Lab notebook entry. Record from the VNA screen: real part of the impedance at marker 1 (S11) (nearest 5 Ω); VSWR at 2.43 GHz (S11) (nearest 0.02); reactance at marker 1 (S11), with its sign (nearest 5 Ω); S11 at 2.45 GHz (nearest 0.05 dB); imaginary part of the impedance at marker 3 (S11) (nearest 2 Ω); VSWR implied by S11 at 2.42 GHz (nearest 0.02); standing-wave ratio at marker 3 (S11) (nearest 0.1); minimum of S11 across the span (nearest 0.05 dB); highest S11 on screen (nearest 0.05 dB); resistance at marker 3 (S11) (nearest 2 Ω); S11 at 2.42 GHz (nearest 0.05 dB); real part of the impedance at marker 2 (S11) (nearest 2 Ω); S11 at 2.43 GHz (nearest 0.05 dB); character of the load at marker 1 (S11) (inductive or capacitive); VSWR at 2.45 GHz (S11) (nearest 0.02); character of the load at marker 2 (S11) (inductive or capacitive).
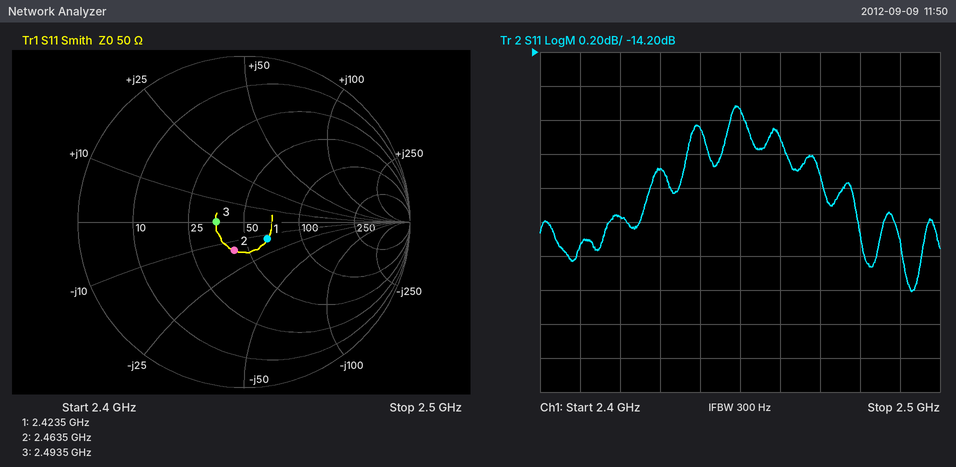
65 Ω
1.44
-15 Ω
-14.55 dB
0 Ω
1.42
1.4
-15.60 dB
-14.50 dB
36 Ω
-15.15 dB
42 Ω
-14.90 dB
capacitive
1.46
capacitive
